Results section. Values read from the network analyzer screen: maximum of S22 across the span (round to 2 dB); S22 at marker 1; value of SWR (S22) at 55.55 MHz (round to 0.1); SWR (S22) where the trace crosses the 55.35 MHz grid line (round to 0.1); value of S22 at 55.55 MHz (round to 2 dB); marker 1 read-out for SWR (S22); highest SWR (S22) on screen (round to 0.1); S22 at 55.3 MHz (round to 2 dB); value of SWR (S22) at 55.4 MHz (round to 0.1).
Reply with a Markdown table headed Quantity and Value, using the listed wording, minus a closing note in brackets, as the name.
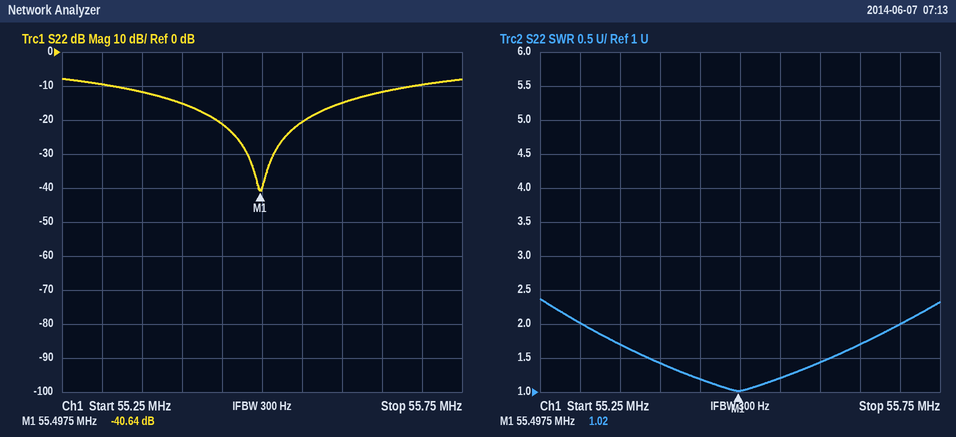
| Quantity | Value |
|---|---|
| maximum of S22 across the span | -8 dB |
| S22 at marker 1 | -40.64 dB |
| value of SWR (S22) at 55.55 MHz | 1.2 |
| SWR (S22) where the trace crosses the 55.35 MHz grid line | 1.7 |
| value of S22 at 55.55 MHz | -20 dB |
| marker 1 read-out for SWR | 1.02 |
| highest SWR (S22) on screen | 2.4 |
| S22 at 55.3 MHz | -10 dB |
| value of SWR (S22) at 55.4 MHz | 1.4 |
